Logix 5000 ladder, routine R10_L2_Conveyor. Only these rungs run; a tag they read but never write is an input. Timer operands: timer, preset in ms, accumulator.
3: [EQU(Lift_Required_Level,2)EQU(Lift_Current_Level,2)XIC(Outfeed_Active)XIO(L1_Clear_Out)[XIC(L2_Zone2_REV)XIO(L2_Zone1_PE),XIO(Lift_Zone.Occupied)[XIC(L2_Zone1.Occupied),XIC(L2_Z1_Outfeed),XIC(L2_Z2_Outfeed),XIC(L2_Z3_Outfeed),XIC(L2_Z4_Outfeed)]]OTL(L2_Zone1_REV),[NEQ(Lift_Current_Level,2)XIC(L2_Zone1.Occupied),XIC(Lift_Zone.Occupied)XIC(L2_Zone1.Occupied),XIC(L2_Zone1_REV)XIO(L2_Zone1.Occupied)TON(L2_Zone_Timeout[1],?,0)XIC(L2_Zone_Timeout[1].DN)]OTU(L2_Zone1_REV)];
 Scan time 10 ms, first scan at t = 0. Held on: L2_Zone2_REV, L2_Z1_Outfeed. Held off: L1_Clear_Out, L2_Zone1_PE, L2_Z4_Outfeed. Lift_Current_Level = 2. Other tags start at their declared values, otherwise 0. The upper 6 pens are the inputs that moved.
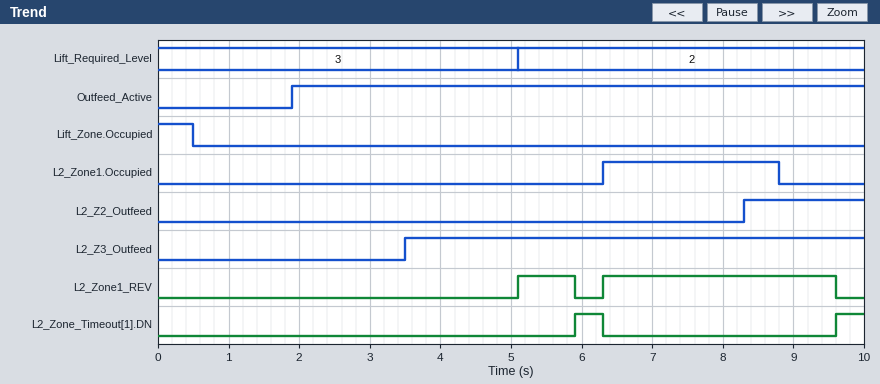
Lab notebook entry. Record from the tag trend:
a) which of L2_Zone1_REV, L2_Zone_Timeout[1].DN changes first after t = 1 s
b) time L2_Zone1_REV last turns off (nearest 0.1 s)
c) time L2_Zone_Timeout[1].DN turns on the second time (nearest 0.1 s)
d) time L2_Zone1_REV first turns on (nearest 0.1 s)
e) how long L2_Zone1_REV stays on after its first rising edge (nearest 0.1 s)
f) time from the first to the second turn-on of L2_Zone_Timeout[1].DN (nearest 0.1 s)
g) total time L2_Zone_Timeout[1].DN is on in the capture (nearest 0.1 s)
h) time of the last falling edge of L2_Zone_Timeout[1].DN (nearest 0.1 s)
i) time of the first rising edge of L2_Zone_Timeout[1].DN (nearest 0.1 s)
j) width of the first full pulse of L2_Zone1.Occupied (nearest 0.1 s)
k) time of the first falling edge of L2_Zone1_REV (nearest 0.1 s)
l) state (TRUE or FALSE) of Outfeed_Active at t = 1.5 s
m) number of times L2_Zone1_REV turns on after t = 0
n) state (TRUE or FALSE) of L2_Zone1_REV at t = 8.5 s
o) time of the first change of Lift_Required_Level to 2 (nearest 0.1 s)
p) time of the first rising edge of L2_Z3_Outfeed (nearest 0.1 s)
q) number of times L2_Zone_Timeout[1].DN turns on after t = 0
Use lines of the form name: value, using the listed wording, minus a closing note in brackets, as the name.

which of L2_Zone1_REV, L2_Zone_Timeout[1].DN changes first after t = 1 s: L2_Zone1_REV
time L2_Zone1_REV last turns off: 9.6 s
time L2_Zone_Timeout[1].DN turns on the second time: 9.6 s
time L2_Zone1_REV first turns on: 5.1 s
how long L2_Zone1_REV stays on after its first rising edge: 0.8 s
time from the first to the second turn-on of L2_Zone_Timeout[1].DN: 3.7 s
total time L2_Zone_Timeout[1].DN is on in the capture: 0.8 s
time of the last falling edge of L2_Zone_Timeout[1].DN: 6.3 s
time of the first rising edge of L2_Zone_Timeout[1].DN: 5.9 s
width of the first full pulse of L2_Zone1.Occupied: 2.5 s
time of the first falling edge of L2_Zone1_REV: 5.9 s
state (TRUE or FALSE) of Outfeed_Active at t = 1.5 s: FALSE
number of times L2_Zone1_REV turns on after t = 0: 2
state (TRUE or FALSE) of L2_Zone1_REV at t = 8.5 s: TRUE
time of the first change of Lift_Required_Level to 2: 5.1 s
time of the first rising edge of L2_Z3_Outfeed: 3.5 s
number of times L2_Zone_Timeout[1].DN turns on after t = 0: 2
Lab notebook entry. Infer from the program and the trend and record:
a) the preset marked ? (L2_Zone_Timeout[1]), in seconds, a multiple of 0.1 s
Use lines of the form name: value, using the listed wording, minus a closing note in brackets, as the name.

the preset marked ? (L2_Zone_Timeout[1]), in seconds, a multiple of 0.1 s: 0.8 s
